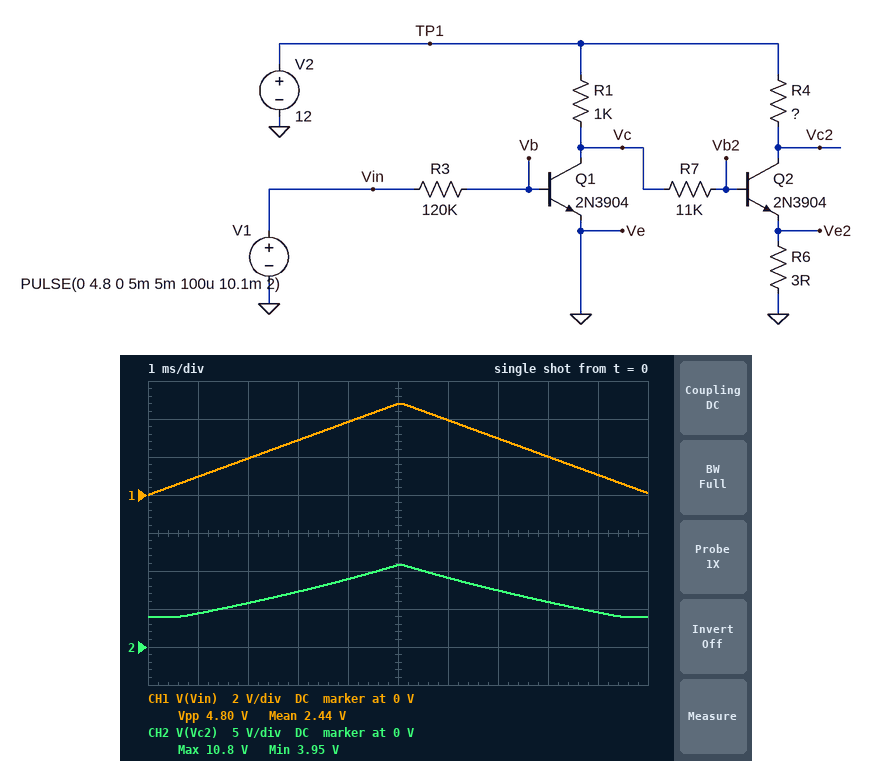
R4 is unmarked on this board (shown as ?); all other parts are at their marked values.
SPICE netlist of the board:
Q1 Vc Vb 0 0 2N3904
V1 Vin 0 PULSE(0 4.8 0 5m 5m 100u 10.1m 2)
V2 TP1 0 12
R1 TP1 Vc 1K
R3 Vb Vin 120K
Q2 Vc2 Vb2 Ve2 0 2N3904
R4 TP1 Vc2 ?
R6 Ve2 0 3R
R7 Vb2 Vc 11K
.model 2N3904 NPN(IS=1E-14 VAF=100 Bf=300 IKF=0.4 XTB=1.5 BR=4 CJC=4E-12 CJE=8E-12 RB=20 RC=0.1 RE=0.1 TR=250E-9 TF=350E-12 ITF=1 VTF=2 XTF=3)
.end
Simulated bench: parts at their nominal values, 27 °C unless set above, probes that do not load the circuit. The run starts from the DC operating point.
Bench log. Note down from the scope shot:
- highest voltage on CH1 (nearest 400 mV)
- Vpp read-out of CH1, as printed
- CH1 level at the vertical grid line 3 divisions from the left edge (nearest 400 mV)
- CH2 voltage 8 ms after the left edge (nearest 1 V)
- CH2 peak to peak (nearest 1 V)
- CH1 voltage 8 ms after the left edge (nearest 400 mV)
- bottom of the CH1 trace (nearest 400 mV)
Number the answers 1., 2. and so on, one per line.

1. 4.8 V
2. 4.80 V
3. 2.8 V
4. 6 V
5. 7 V
6. 2.0 V
7. 0 V
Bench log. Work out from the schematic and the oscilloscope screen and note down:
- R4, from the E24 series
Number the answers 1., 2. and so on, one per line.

1. 43 Ω
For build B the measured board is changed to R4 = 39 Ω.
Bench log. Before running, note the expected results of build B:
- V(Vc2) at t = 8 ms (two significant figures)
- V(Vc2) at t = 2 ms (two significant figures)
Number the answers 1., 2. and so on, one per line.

1. 6.5 V
2. 6.3 V
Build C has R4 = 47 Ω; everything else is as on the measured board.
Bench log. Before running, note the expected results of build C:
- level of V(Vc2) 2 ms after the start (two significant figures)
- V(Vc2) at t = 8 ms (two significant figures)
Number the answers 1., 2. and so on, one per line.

1. 5.2 V
2. 5.4 V
